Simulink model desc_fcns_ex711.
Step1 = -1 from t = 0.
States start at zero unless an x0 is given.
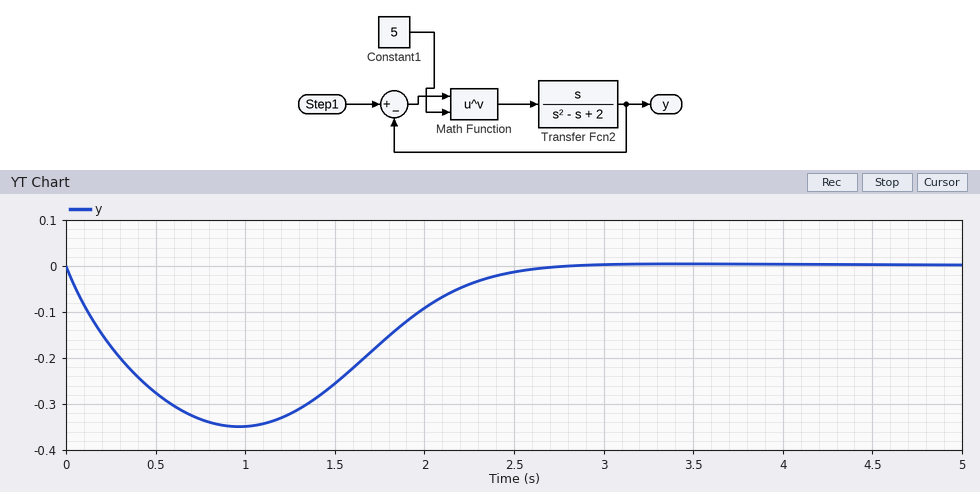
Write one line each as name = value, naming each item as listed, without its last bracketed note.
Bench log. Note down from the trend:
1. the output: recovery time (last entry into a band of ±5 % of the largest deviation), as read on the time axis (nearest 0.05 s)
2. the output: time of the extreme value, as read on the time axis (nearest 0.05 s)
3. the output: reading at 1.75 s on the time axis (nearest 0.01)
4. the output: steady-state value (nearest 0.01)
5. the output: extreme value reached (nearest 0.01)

the output: recovery time (last entry into a band of ±5 % of the largest deviation), as read on the time axis = 2.45 s
the output: time of the extreme value, as read on the time axis = 0.95 s
the output: reading at 1.75 s on the time axis = -0.17
the output: steady-state value = 0.00
the output: extreme value reached = -0.35
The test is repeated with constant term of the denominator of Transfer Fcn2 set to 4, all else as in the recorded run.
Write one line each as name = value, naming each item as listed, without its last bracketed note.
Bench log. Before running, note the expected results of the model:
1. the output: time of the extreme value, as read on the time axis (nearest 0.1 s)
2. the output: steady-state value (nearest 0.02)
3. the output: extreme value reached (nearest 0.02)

the output: time of the extreme value, as read on the time axis = 0.7 s
the output: steady-state value = 0.00
the output: extreme value reached = -0.26
